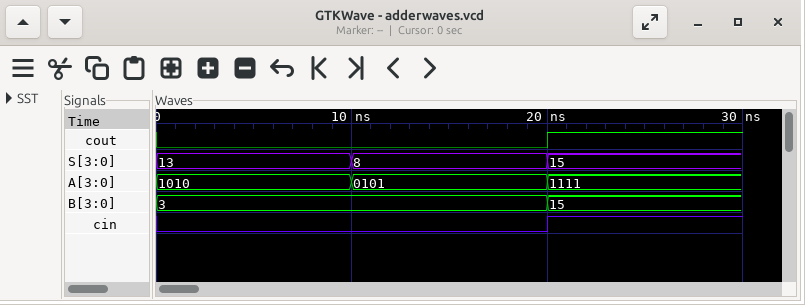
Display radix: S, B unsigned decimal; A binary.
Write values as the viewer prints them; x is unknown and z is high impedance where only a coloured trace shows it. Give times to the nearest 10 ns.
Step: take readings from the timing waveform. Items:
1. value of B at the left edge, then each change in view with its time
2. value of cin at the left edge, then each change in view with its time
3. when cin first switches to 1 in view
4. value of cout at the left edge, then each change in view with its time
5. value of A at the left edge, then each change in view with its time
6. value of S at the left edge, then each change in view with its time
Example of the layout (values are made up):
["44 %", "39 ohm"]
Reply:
["3, 15 at 20 ns", "0, 1 at 20 ns", "20 ns", "0, 1 at 20 ns", "1010, 0101 at 10 ns, 1111 at 20 ns", "13, 8 at 10 ns, 15 at 20 ns"]
